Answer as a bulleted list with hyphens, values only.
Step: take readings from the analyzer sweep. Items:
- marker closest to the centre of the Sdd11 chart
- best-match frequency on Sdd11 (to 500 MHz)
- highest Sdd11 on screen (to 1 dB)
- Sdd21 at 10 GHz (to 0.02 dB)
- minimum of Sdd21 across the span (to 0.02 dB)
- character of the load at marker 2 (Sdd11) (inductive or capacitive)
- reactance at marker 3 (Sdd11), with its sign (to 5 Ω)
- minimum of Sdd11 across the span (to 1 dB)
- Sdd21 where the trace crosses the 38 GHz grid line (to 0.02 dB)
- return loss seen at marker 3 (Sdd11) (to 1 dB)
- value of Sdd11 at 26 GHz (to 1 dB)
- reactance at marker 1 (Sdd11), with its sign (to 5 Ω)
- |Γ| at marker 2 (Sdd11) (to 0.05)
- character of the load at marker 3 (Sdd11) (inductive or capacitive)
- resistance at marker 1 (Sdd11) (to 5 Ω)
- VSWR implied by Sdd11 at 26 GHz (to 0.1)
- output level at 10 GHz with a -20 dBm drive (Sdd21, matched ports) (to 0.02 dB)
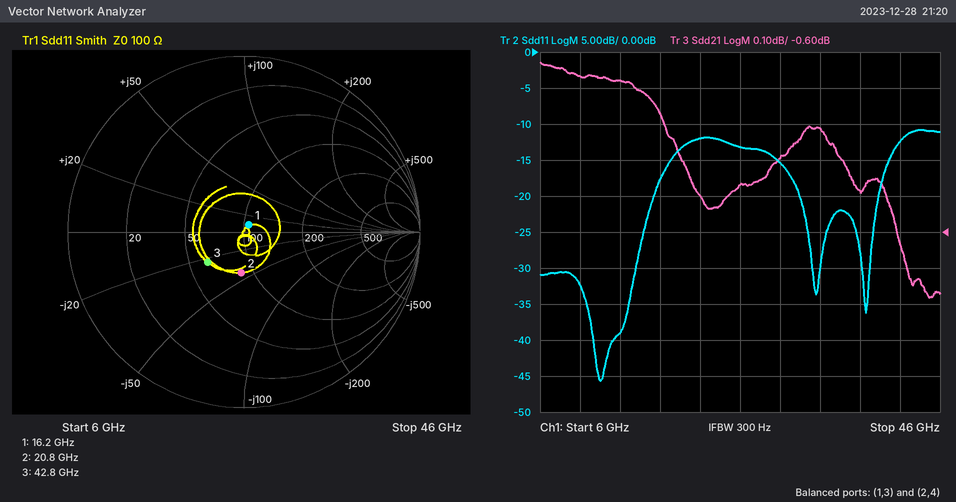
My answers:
- marker 1
- 12.0 GHz
- -11 dB
- -0.16 dB
- -0.78 dB
- capacitive
- -25 Ω
- -46 dB
- -0.48 dB
- 11 dB
- -13 dB
- +10 Ω
- 0.25
- capacitive
- 105 Ω
- 1.6
- -20.16 dBm
